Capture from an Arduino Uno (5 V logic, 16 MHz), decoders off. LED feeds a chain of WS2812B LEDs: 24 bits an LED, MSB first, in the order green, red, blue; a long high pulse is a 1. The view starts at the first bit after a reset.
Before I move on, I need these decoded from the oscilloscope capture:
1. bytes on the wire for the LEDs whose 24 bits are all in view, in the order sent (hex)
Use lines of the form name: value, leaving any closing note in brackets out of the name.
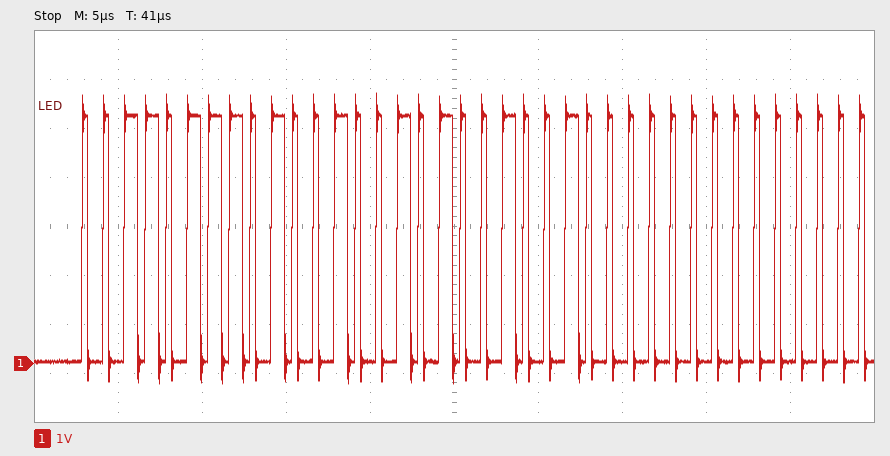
bytes on the wire for the LEDs whose 24 bits are all in view, in the order sent: 37 49 49
